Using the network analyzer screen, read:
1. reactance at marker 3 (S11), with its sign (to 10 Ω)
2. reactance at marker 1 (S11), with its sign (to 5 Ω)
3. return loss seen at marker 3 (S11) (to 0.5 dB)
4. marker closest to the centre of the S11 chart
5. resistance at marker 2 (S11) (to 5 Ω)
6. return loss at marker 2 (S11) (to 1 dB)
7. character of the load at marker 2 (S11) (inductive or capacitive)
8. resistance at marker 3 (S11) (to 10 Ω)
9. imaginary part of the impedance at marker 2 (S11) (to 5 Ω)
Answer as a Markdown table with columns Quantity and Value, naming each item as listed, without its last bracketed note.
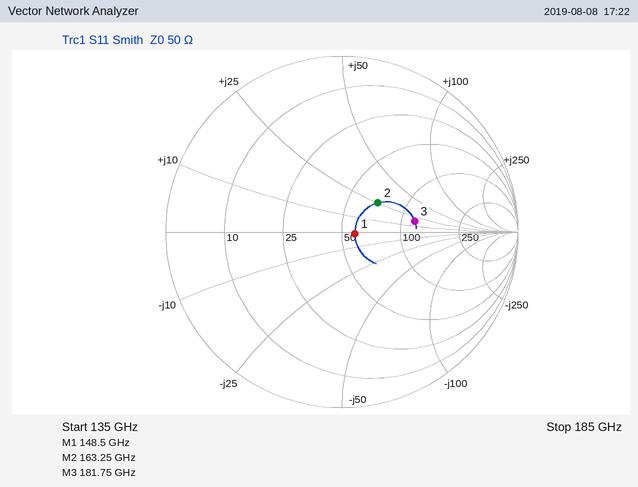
| Quantity | Value |
|---|---|
| reactance at marker 3 (S11), with its sign | +20 Ω |
| reactance at marker 1 (S11), with its sign | 0 Ω |
| return loss seen at marker 3 (S11) | 7.5 dB |
| marker closest to the centre of the S11 chart | marker 1 |
| resistance at marker 2 (S11) | 70 Ω |
| return loss at marker 2 (S11) | 12 dB |
| character of the load at marker 2 (S11) | inductive |
| resistance at marker 3 (S11) | 120 Ω |
| imaginary part of the impedance at marker 2 (S11) | +25 Ω |
